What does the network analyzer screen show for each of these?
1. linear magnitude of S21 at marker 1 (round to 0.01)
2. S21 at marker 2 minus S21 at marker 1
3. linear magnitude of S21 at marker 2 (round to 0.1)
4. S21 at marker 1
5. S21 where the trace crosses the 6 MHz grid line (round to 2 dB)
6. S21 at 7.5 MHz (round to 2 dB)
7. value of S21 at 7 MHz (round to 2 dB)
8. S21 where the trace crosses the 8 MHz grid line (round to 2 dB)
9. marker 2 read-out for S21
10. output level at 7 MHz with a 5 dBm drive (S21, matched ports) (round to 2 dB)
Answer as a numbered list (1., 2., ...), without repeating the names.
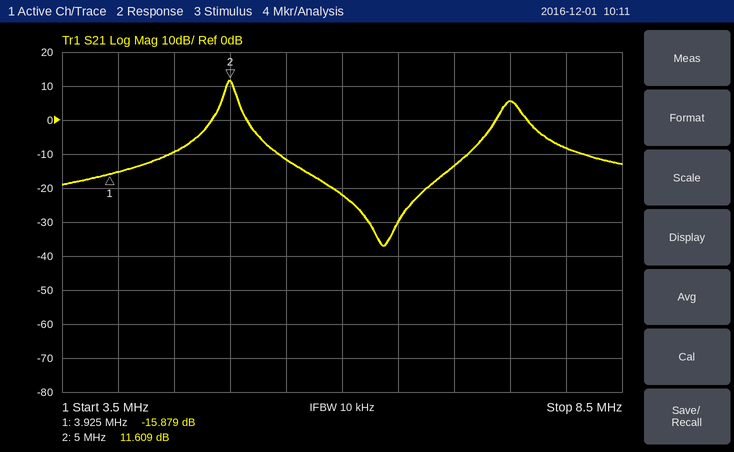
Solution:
1. 0.16
2. 27.488 dB
3. 3.8
4. -15.879 dB
5. -22 dB
6. 6 dB
7. -14 dB
8. -8 dB
9. 11.609 dB
10. -8 dBm
